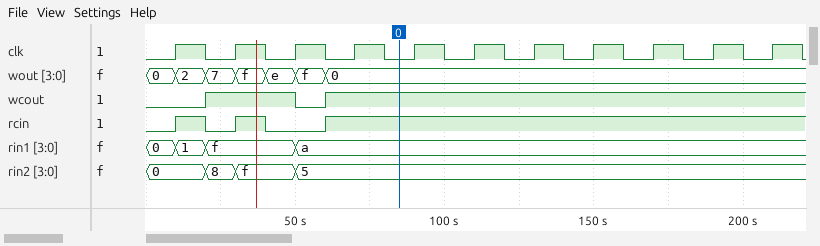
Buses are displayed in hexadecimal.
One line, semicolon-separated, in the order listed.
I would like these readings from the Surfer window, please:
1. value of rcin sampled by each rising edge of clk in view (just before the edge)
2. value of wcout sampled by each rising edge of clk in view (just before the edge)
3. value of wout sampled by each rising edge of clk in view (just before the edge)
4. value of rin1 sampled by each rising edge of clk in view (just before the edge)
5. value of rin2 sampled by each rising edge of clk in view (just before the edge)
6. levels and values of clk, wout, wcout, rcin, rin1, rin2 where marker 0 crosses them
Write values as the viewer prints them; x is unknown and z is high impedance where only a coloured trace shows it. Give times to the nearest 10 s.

0 0 0 1 1 1 1 1 1 1 1; 0 1 1 1 1 1 1 1 1 1 1; 0, 7, e, 0, 0, 0, 0, 0, 0, 0, 0; 0, f, f, a, a, a, a, a, a, a, a; 0, 8, f, 5, 5, 5, 5, 5, 5, 5, 5; clk=0, wout=0, wcout=1, rcin=1, rin1=a, rin2=5
